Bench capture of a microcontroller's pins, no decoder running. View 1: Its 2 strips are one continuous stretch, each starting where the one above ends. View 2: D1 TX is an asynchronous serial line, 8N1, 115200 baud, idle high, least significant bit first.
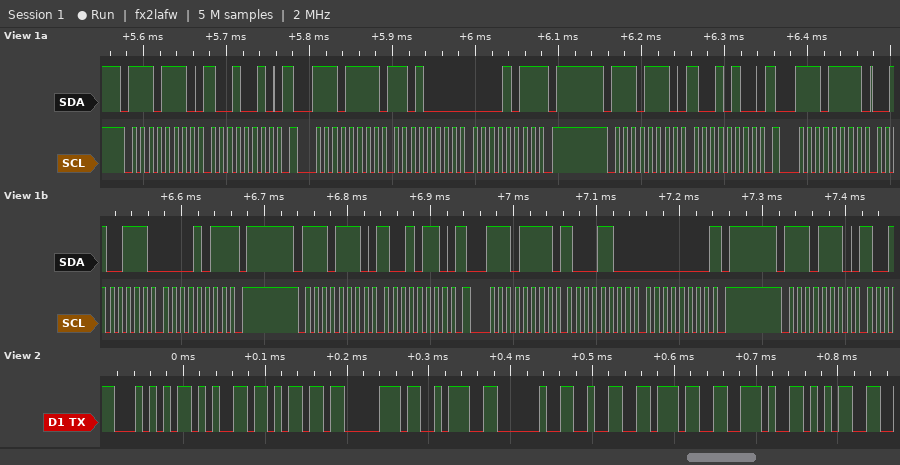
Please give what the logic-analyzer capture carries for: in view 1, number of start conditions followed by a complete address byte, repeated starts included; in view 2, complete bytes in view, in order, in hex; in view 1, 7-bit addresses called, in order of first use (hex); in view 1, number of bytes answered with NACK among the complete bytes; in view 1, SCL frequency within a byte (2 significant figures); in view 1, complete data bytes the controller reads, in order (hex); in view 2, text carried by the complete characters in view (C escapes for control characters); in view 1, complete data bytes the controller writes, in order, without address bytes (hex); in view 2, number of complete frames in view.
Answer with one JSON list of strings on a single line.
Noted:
["7", "54 65 6D 70 3A 20 32 37 2E 35", "0x77", "3", "100 kHz", "D0 0B 27 0B 8C 00", "\"Temp: 27.5\"", "92 94 96", "10"]
